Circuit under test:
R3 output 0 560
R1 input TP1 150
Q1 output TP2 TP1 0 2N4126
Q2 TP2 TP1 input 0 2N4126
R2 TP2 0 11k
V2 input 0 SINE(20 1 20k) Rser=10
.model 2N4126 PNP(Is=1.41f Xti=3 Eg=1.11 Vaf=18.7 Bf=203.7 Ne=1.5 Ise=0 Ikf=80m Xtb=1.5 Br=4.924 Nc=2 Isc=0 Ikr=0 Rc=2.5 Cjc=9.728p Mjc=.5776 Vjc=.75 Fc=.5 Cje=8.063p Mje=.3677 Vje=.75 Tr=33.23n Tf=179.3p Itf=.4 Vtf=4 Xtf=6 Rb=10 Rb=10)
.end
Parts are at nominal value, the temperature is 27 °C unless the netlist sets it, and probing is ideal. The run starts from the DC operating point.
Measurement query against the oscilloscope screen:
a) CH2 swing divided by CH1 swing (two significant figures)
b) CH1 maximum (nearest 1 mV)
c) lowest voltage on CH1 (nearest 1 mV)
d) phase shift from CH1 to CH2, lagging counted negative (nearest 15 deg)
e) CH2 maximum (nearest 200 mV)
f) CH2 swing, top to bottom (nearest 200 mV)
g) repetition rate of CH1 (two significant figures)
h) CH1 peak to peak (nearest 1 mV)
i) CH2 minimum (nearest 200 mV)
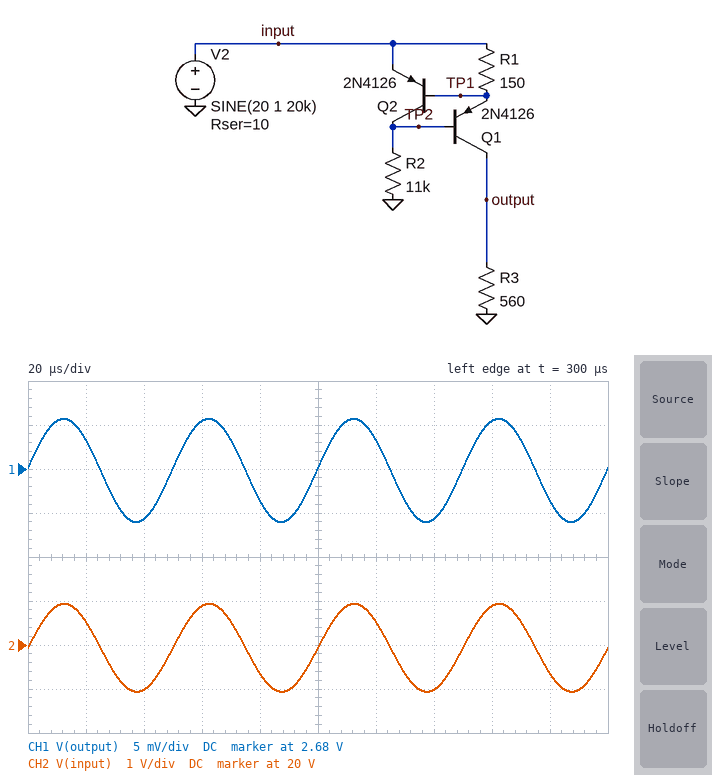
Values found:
170
2.686 V
2.674 V
0 deg
21.0 V
2.0 V
20 kHz
12 mV
19.0 V
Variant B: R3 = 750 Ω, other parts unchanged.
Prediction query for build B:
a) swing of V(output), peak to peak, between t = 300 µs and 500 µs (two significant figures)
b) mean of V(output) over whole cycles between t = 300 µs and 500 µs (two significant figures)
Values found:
16 mV
3.6 V
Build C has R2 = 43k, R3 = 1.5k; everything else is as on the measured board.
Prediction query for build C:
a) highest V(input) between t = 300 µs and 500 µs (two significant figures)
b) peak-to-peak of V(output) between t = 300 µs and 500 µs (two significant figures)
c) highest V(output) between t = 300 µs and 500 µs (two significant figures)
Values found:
21 V
31 mV
6.8 V
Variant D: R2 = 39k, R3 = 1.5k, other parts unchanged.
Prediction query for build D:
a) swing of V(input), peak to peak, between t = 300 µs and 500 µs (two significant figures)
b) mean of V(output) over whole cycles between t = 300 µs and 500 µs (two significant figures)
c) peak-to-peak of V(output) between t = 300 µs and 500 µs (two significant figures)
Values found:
2.0 V
6.8 V
31 mV
